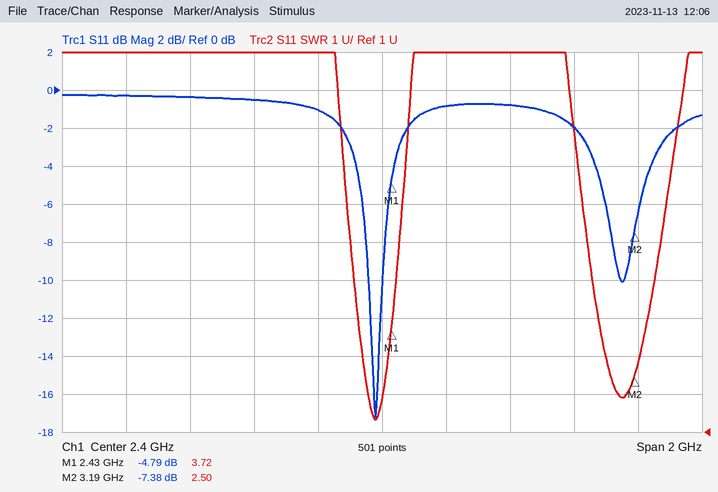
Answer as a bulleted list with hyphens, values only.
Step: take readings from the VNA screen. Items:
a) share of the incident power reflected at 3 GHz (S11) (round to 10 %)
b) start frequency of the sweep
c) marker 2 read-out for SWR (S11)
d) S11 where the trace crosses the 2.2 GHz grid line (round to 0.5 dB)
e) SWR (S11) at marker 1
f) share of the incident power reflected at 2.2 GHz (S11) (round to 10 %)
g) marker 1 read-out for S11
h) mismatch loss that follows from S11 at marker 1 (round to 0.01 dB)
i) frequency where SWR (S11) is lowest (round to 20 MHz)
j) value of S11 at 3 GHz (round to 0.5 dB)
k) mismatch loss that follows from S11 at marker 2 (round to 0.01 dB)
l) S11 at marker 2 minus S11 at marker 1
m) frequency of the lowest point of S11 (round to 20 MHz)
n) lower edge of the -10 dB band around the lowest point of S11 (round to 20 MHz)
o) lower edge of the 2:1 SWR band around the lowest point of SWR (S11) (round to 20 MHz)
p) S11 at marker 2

- 60 %
- 1.4 GHz
- 2.50
- -1.0 dB
- 3.72
- 80 %
- -4.79 dB
- 1.75 dB
- 2.38 GHz
- -2.0 dB
- 0.88 dB
- -2.59 dB
- 2.38 GHz
- 2.36 GHz
- 2.36 GHz
- -7.38 dB
